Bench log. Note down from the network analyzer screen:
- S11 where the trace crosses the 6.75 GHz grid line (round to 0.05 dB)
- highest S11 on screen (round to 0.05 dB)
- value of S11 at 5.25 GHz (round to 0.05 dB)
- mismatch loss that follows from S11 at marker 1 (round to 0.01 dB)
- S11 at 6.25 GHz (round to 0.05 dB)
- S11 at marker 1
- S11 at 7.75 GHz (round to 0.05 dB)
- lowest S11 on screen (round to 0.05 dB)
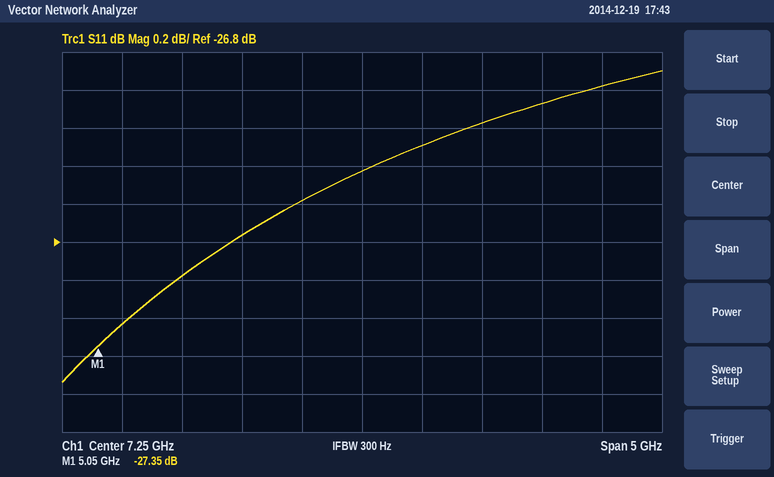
-26.60 dB
-25.90 dB
-27.25 dB
0.01 dB
-26.75 dB
-27.35 dB
-26.30 dB
-27.55 dB
